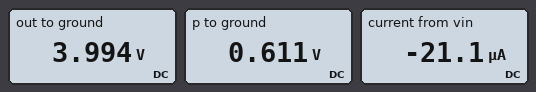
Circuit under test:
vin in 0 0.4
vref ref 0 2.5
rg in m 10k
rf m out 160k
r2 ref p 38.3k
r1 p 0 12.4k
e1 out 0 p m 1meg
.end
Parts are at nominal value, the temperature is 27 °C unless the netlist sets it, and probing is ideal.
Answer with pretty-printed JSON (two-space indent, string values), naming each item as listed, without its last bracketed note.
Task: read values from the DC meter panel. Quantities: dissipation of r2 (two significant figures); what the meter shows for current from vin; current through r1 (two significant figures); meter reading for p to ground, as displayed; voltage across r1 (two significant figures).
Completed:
{
  "dissipation of r2": "93 µW",
  "what the meter shows for current from vin": "-21.1 µA",
  "current through r1": "49 µA",
  "meter reading for p to ground, as displayed": "0.611 V",
  "voltage across r1": "610 mV"
}
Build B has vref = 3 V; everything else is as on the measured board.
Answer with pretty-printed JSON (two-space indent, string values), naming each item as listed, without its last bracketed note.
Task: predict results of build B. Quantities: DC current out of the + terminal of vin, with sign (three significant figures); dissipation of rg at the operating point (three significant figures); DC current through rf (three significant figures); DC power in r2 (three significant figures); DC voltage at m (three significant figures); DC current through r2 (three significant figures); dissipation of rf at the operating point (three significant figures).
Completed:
{
  "DC current out of the + terminal of vin, with sign": "-33.4 µA",
  "dissipation of rg at the operating point": "11.1 µW",
  "DC current through rf": "33.4 µA",
  "DC power in r2": "134 µW",
  "DC voltage at m": "734 mV",
  "DC current through r2": "59.2 µA",
  "dissipation of rf at the operating point": "178 µW"
}
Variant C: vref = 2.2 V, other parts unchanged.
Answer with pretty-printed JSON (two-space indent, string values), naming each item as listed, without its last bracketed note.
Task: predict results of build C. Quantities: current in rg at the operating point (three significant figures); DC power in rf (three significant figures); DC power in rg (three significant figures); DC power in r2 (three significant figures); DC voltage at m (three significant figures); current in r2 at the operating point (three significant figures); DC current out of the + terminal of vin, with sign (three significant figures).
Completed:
{
  "current in rg at the operating point": "13.8 µA",
  "DC power in rf": "30.5 µW",
  "DC power in rg": "1.91 µW",
  "DC power in r2": "72.1 µW",
  "DC voltage at m": "538 mV",
  "current in r2 at the operating point": "43.4 µA",
  "DC current out of the + terminal of vin, with sign": "-13.8 µA"
}
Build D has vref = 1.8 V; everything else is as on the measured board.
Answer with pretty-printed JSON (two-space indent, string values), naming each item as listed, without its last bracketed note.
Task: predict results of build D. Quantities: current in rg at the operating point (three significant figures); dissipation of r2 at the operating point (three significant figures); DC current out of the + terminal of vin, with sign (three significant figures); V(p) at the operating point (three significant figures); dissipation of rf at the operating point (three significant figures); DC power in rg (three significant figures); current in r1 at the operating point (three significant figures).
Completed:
{
  "current in rg at the operating point": "4.02 µA",
  "dissipation of r2 at the operating point": "48.3 µW",
  "DC current out of the + terminal of vin, with sign": "-4.02 µA",
  "V(p) at the operating point": "440 mV",
  "dissipation of rf at the operating point": "2.59 µW",
  "DC power in rg": "162 nW",
  "current in r1 at the operating point": "35.5 µA"
}
